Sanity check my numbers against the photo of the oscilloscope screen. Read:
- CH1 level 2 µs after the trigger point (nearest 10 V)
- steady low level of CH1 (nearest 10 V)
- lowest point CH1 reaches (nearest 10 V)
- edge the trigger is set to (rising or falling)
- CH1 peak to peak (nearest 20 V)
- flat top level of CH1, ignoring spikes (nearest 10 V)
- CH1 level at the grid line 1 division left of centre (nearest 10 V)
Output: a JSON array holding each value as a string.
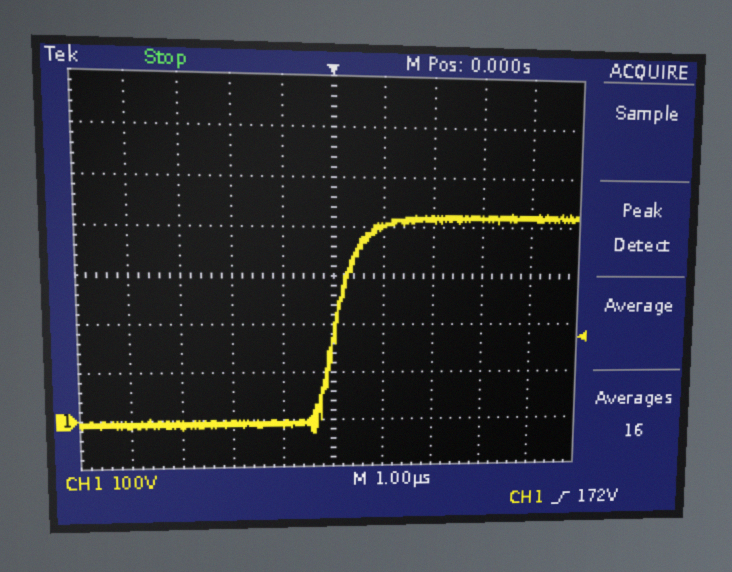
["420 V", "-10 V", "-30 V", "rising", "460 V", "420 V", "-10 V"]
